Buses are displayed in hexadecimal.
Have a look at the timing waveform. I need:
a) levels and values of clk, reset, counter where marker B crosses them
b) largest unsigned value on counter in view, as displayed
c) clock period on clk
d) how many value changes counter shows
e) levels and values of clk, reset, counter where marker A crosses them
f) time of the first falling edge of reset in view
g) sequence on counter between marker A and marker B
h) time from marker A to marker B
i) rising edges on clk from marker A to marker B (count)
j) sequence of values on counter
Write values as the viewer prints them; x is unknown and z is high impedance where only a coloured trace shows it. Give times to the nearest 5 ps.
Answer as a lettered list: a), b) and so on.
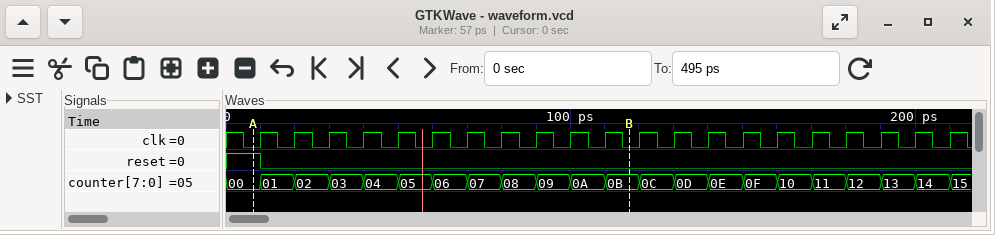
a) clk=0, reset=0, counter=0B
b) 15
c) 10 ps
d) 21
e) clk=0, reset=1, counter=00
f) 10 ps
g) 00, 01, 02, 03, 04, 05, 06, 07, 08, 09, 0A, 0B
h) 110 ps
i) 11
j) 00, 01, 02, 03, 04, 05, 06, 07, 08, 09, 0A, 0B, 0C, 0D, 0E, 0F, 10, 11, 12, 13, 14, 15
